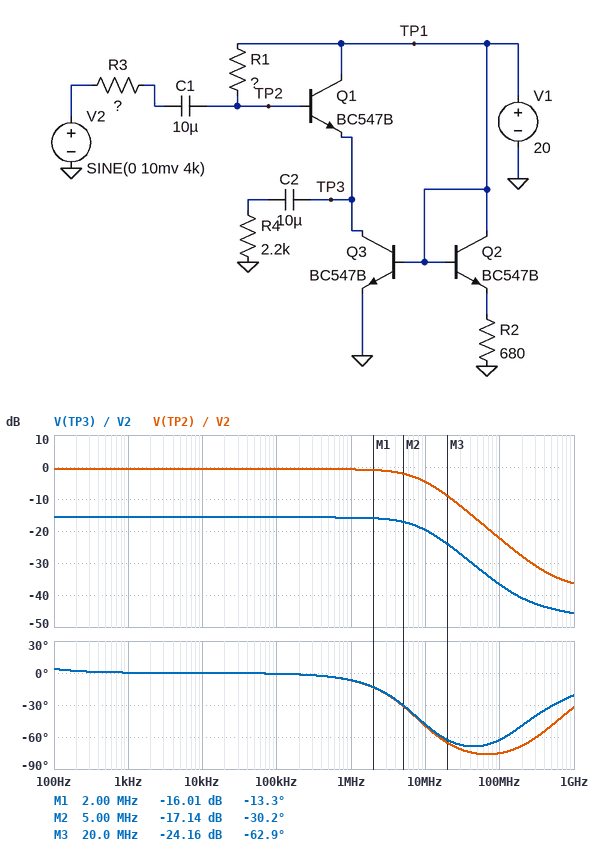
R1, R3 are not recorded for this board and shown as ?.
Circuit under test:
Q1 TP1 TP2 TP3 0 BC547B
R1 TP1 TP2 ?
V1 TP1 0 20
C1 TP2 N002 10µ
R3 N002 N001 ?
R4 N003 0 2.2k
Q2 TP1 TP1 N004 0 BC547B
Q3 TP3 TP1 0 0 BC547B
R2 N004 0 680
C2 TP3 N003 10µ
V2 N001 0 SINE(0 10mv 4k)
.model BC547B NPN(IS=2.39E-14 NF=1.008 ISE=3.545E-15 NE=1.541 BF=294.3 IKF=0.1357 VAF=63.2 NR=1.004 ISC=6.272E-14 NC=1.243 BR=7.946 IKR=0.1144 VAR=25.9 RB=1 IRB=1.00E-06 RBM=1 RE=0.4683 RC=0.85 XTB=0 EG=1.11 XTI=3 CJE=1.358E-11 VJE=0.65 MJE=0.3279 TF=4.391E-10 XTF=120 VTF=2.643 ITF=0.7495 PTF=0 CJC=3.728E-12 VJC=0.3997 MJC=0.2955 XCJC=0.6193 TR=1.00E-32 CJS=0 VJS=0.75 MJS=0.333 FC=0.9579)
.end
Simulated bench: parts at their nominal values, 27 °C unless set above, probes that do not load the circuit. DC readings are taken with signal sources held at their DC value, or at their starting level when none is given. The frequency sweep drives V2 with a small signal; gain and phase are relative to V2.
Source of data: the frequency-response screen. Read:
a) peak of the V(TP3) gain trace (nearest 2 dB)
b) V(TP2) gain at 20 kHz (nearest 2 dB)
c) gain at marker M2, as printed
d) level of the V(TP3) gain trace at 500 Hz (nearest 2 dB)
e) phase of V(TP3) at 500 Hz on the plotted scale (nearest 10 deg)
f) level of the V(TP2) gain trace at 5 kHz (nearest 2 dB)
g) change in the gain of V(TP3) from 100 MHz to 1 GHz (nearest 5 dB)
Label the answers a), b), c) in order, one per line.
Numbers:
a) -16 dB
b) 0 dB
c) -17.14 dB
d) -16 dB
e) 0 deg
f) 0 dB
g) -10 dB
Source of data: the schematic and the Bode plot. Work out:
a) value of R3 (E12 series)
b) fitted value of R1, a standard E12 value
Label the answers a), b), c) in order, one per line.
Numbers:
a) 180 Ω
b) 820 kΩ
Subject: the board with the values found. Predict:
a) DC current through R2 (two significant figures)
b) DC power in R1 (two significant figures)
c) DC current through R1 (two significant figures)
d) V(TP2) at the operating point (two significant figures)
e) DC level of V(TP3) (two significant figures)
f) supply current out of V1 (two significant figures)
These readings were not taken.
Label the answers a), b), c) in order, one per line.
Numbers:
a) 28 mA
b) 210 µW
c) 16 µA
d) 6.8 V
e) 6.1 V
f) 13 A
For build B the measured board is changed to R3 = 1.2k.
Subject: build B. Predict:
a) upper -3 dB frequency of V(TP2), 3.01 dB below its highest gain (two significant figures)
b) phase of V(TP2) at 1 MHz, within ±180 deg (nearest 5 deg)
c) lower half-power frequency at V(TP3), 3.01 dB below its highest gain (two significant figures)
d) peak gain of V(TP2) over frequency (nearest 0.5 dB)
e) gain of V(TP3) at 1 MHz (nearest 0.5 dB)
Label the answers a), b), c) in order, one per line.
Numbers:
a) 1.8 MHz
b) -30 deg
c) 4.7 Hz
d) -4.0 dB
e) -20.0 dB
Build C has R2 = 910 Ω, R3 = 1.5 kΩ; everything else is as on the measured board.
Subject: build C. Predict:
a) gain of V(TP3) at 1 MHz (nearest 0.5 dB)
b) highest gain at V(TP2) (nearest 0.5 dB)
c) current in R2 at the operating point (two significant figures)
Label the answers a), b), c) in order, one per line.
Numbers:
a) -21.0 dB
b) -4.5 dB
c) 21 mA
